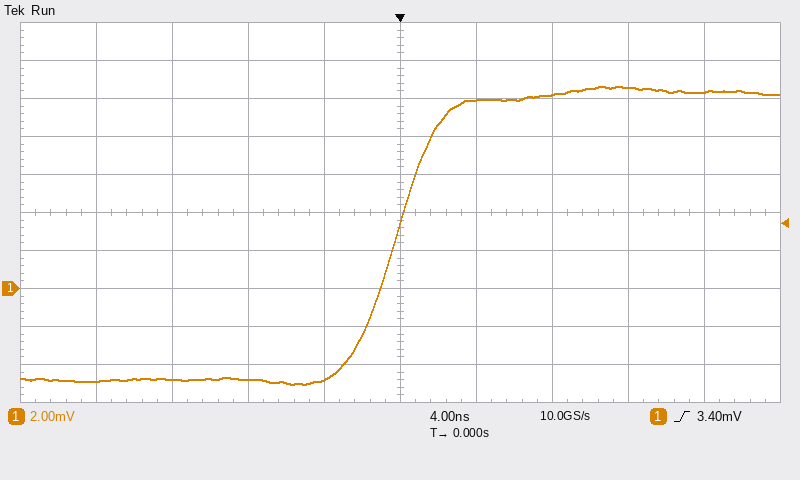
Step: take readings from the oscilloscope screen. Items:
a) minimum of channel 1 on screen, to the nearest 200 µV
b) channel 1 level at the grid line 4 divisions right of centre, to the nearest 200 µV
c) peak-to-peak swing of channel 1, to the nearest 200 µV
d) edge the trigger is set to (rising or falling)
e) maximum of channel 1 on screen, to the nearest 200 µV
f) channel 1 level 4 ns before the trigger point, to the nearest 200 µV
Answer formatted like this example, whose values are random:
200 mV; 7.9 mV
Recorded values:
-5.0 mV; 10.4 mV; 15.6 mV; rising; 10.6 mV; -4.8 mV
